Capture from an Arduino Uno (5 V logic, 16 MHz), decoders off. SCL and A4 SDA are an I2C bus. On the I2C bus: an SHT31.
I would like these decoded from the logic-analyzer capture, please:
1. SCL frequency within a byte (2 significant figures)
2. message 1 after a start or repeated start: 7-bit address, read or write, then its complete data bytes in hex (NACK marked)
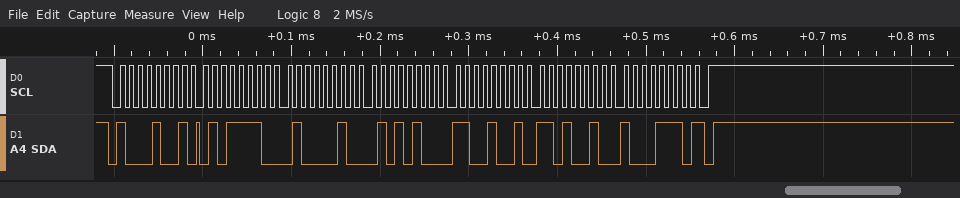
100 kHz
0x44 read: 5E 42 54 C9 D2 8E NACK
